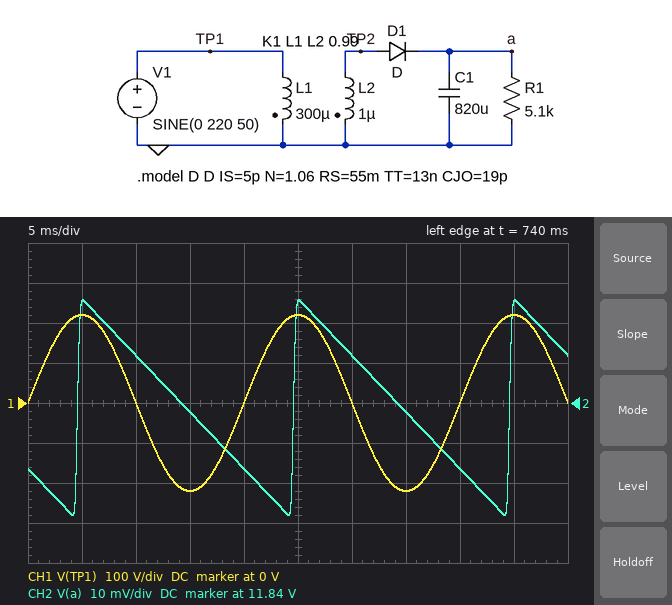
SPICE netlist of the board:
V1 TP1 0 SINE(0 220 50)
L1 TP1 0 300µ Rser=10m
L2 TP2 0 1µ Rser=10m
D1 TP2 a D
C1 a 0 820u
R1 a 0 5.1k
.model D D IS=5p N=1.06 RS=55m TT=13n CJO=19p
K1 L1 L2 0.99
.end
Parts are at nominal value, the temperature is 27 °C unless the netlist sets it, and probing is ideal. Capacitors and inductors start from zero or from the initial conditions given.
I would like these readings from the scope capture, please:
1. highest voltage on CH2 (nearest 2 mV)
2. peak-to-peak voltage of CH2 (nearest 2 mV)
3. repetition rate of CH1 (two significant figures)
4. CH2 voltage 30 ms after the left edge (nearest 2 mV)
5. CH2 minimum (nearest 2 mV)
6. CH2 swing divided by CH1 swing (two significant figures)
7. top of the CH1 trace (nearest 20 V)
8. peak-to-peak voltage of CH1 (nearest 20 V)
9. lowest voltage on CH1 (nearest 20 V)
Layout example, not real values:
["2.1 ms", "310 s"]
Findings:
["11.866 V", "54 mV", "50 Hz", "11.852 V", "11.812 V", "0.00012", "220 V", "440 V", "-220 V"]
